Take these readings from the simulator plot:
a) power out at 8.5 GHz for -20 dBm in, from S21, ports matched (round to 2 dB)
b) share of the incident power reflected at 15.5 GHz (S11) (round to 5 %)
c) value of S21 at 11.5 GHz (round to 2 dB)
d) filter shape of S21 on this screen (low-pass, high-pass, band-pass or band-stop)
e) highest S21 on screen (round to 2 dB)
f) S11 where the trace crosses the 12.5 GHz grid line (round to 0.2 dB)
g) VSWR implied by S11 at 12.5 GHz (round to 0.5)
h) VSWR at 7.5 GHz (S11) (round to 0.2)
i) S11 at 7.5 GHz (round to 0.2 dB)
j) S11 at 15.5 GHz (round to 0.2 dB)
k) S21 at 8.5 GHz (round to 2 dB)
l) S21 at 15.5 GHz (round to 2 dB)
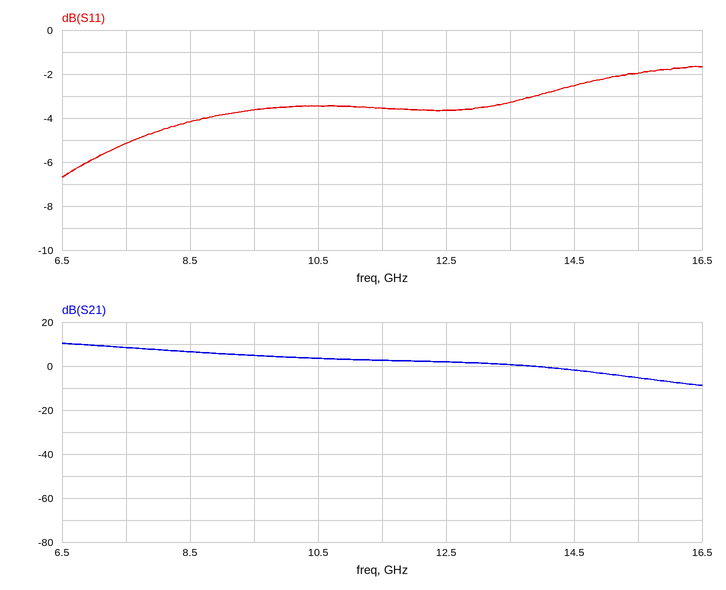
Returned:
-14 dBm
65 %
2 dB
low-pass
10 dB
-3.6 dB
5.0
3.4
-5.2 dB
-2.0 dB
6 dB
-6 dB
